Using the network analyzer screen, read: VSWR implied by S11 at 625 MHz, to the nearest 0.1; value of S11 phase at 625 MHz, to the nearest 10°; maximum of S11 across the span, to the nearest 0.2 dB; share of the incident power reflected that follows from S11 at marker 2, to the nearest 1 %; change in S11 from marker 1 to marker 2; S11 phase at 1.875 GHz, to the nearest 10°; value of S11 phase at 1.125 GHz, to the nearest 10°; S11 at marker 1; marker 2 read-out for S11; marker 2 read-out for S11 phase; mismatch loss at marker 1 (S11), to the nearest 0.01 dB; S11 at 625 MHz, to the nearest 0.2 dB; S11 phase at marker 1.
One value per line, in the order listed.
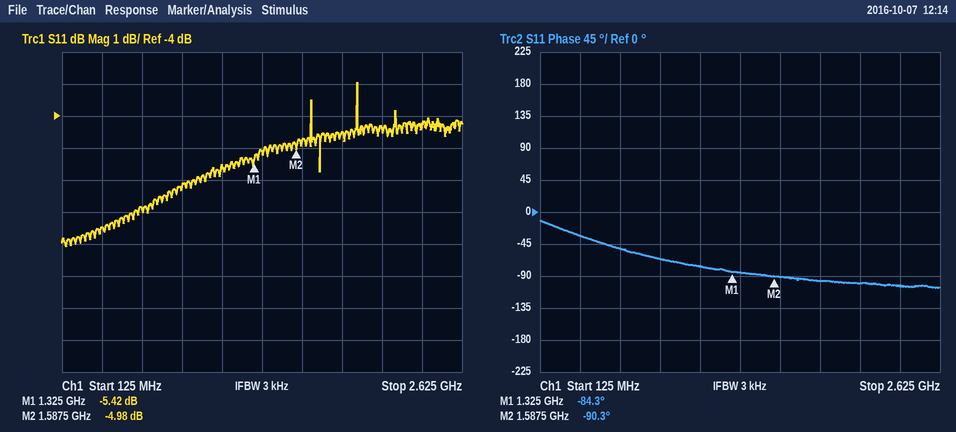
2.6
-50°
-3.0 dB
32 %
0.44 dB
-100°
-80°
-5.42 dB
-4.98 dB
-90.3°
1.47 dB
-7.0 dB
-84.3°
